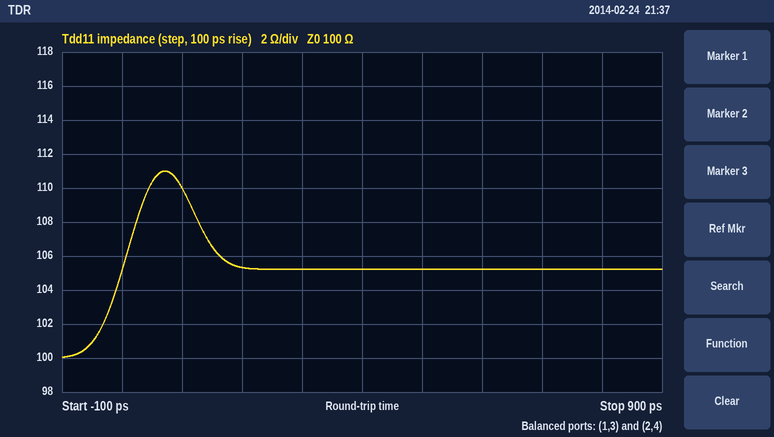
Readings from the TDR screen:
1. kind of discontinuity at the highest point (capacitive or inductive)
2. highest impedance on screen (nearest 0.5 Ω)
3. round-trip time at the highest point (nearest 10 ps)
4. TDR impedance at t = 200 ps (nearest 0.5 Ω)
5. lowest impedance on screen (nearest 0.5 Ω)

inductive
111.0 Ω
70 ps
105.5 Ω
100.0 Ω
